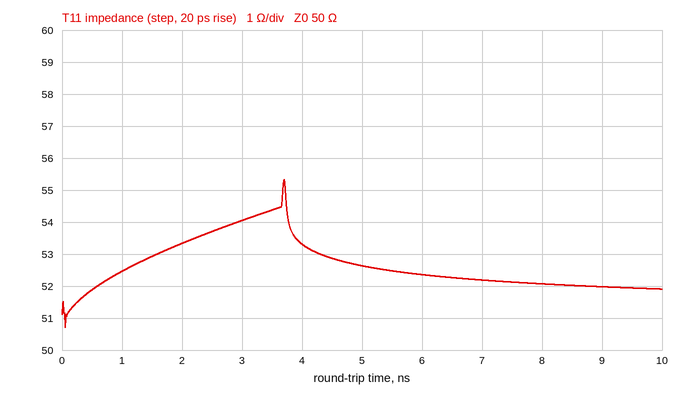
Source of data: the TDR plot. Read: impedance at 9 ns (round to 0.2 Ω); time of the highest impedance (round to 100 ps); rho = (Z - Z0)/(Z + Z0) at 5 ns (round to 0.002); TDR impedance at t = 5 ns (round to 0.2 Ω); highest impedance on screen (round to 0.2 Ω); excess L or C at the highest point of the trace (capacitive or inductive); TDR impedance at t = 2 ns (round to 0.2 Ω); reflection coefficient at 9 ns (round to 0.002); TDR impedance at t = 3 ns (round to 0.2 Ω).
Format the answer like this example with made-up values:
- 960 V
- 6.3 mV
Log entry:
- 52.0 Ω
- 3.7 ns
- +0.026
- 52.6 Ω
- 55.4 Ω
- inductive
- 53.4 Ω
- +0.020
- 54.0 Ω
